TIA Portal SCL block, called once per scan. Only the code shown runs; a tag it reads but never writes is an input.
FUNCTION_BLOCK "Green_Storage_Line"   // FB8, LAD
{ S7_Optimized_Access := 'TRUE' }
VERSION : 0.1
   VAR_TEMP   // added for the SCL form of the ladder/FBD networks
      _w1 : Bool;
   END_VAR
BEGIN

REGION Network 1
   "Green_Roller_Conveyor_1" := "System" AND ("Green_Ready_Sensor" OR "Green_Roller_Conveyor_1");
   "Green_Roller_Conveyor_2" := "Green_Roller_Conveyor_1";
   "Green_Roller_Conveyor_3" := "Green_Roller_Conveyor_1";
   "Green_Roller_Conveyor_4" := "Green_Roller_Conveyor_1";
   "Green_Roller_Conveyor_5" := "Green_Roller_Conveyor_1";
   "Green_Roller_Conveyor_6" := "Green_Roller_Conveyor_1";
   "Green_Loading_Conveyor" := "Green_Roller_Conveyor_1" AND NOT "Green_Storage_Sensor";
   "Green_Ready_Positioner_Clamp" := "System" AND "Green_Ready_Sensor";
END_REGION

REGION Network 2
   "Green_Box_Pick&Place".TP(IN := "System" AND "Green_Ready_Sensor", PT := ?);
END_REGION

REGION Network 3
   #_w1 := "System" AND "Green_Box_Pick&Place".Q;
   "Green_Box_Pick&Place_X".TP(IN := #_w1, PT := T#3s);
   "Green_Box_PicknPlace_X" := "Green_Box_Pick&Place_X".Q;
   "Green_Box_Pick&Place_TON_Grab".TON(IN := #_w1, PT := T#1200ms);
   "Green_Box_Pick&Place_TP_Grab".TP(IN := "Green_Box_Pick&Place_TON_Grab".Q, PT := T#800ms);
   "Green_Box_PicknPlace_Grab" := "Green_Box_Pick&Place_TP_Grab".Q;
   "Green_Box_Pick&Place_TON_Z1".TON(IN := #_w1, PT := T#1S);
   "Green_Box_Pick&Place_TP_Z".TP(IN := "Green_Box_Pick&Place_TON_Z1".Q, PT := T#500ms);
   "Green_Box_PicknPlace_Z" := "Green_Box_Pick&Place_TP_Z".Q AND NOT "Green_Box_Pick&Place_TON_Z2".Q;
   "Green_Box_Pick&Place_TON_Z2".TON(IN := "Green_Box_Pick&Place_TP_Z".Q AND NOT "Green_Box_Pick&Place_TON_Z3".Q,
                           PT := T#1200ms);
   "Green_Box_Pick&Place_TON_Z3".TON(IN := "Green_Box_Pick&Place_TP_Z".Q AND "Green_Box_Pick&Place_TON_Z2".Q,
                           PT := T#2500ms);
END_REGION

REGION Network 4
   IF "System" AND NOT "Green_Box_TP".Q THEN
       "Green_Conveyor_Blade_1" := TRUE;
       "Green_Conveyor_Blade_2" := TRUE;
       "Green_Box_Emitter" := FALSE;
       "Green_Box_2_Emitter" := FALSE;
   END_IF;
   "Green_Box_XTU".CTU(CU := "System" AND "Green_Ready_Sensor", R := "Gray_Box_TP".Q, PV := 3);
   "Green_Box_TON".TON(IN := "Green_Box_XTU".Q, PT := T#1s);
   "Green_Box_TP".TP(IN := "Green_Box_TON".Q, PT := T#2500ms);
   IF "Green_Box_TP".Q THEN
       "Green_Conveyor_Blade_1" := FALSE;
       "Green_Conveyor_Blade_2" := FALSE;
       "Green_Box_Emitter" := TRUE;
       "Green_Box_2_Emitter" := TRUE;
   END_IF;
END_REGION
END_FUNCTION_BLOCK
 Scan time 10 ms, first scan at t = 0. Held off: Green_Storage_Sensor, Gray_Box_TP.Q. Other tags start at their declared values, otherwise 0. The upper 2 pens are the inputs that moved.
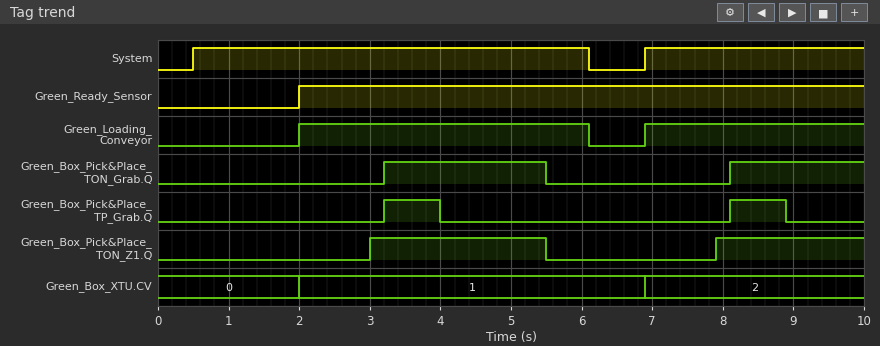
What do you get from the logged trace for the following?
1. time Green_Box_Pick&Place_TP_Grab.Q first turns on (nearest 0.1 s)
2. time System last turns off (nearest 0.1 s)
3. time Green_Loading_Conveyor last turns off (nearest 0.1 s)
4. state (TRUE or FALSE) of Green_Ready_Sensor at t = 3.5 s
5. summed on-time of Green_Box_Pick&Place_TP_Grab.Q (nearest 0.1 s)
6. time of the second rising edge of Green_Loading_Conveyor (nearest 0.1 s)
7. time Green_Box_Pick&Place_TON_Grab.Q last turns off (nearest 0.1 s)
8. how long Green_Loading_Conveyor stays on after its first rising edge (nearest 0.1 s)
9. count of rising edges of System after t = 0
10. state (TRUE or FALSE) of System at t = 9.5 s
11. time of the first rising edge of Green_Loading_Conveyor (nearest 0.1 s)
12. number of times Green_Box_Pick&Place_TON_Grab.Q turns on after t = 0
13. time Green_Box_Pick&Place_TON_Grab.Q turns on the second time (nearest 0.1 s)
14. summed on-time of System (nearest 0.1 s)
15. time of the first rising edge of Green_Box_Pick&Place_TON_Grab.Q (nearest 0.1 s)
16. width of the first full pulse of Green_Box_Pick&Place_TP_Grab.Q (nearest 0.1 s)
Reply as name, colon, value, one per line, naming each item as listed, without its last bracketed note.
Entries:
time Green_Box_Pick&Place_TP_Grab.Q first turns on: 3.2 s
time System last turns off: 6.1 s
time Green_Loading_Conveyor last turns off: 6.1 s
state (TRUE or FALSE) of Green_Ready_Sensor at t = 3.5 s: TRUE
summed on-time of Green_Box_Pick&Place_TP_Grab.Q: 1.6 s
time of the second rising edge of Green_Loading_Conveyor: 6.9 s
time Green_Box_Pick&Place_TON_Grab.Q last turns off: 5.5 s
how long Green_Loading_Conveyor stays on after its first rising edge: 4.1 s
count of rising edges of System after t = 0: 2
state (TRUE or FALSE) of System at t = 9.5 s: TRUE
time of the first rising edge of Green_Loading_Conveyor: 2.0 s
number of times Green_Box_Pick&Place_TON_Grab.Q turns on after t = 0: 2
time Green_Box_Pick&Place_TON_Grab.Q turns on the second time: 8.1 s
summed on-time of System: 8.7 s
time of the first rising edge of Green_Box_Pick&Place_TON_Grab.Q: 3.2 s
width of the first full pulse of Green_Box_Pick&Place_TP_Grab.Q: 0.8 s
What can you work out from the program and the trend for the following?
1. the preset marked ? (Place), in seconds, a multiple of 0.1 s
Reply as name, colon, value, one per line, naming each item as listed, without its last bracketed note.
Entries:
the preset marked ? (Place), in seconds, a multiple of 0.1 s: 3.5 s
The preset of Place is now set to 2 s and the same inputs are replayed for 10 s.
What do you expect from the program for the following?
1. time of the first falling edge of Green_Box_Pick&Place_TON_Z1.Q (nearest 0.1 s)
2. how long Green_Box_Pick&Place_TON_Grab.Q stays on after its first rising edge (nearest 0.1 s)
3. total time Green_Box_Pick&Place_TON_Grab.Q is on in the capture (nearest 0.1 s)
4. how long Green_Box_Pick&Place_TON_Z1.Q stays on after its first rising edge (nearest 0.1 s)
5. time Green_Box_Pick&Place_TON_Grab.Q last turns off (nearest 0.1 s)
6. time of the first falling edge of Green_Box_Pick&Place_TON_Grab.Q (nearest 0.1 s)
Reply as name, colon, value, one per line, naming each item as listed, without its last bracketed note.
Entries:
time of the first falling edge of Green_Box_Pick&Place_TON_Z1.Q: 4.0 s
how long Green_Box_Pick&Place_TON_Grab.Q stays on after its first rising edge: 0.8 s
total time Green_Box_Pick&Place_TON_Grab.Q is on in the capture: 1.6 s
how long Green_Box_Pick&Place_TON_Z1.Q stays on after its first rising edge: 1.0 s
time Green_Box_Pick&Place_TON_Grab.Q last turns off: 8.9 s
time of the first falling edge of Green_Box_Pick&Place_TON_Grab.Q: 4.0 s
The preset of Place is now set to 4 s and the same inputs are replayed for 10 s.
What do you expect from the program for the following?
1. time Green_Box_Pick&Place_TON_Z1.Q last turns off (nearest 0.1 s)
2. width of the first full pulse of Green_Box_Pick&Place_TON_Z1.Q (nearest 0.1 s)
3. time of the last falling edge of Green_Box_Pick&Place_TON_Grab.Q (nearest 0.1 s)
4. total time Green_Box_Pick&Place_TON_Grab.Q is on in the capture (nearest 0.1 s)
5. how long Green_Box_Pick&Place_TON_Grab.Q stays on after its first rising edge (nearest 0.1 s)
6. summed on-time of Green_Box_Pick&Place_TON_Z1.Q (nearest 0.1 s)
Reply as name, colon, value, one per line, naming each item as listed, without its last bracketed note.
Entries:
time Green_Box_Pick&Place_TON_Z1.Q last turns off: 6.0 s
width of the first full pulse of Green_Box_Pick&Place_TON_Z1.Q: 3.0 s
time of the last falling edge of Green_Box_Pick&Place_TON_Grab.Q: 6.0 s
total time Green_Box_Pick&Place_TON_Grab.Q is on in the capture: 4.7 s
how long Green_Box_Pick&Place_TON_Grab.Q stays on after its first rising edge: 2.8 s
summed on-time of Green_Box_Pick&Place_TON_Z1.Q: 5.1 s
